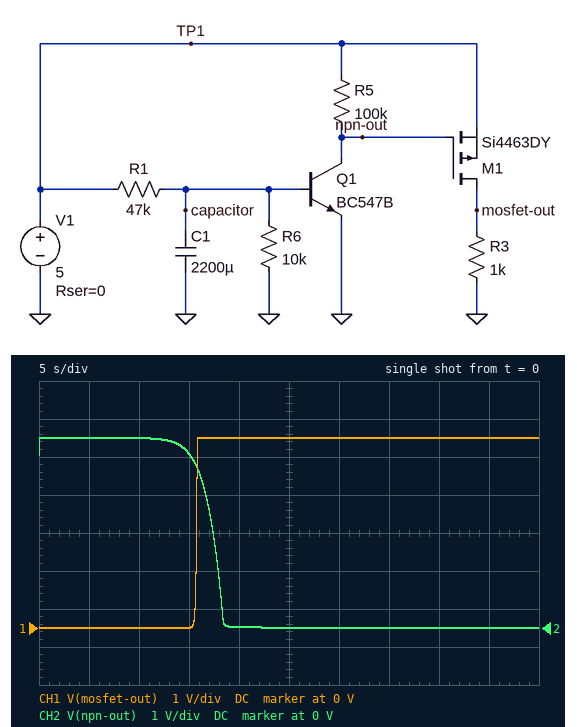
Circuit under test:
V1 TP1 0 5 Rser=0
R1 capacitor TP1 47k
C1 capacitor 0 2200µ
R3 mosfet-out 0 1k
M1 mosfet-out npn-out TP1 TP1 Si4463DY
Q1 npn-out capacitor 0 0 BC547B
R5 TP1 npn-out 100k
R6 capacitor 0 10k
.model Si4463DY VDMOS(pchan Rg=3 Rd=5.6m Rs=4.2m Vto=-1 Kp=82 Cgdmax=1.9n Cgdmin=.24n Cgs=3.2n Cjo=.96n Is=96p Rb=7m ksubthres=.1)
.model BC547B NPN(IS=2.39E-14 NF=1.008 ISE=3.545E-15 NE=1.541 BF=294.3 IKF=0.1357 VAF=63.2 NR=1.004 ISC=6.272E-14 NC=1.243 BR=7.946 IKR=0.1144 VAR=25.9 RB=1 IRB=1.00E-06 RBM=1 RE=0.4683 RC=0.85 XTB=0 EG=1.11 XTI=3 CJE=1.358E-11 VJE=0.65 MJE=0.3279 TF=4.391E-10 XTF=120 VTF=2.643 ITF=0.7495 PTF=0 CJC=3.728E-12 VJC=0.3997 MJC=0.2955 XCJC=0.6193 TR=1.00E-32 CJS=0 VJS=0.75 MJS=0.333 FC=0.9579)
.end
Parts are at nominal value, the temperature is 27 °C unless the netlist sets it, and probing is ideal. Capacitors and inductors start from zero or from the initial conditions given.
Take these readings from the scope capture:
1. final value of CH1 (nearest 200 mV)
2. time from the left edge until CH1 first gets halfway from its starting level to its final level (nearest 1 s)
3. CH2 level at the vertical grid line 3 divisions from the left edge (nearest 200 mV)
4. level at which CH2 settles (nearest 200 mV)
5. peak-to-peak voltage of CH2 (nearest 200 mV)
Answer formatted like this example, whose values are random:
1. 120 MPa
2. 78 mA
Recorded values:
1. 5.0 V
2. 16 s
3. 4.6 V
4. 0 V
5. 5.0 V
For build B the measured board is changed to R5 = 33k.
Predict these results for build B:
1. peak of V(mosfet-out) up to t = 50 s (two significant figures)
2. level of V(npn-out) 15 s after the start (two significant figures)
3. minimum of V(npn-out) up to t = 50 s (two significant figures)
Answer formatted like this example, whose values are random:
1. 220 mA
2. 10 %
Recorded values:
1. 5.0 V
2. 4.9 V
3. 20 mV
